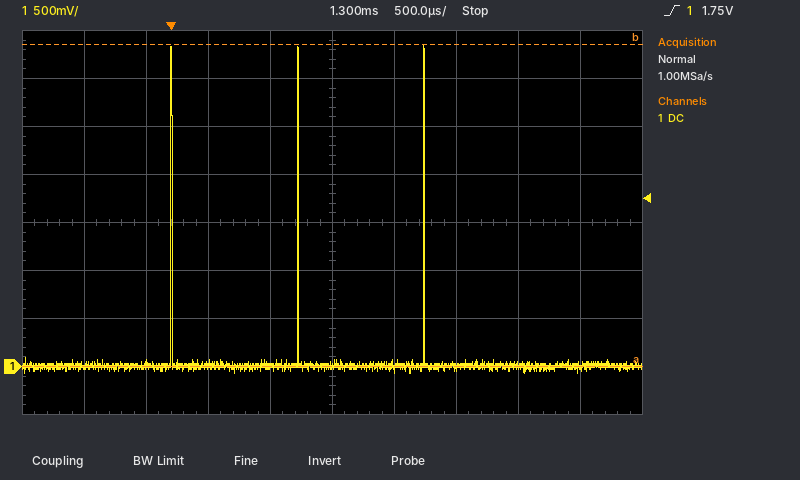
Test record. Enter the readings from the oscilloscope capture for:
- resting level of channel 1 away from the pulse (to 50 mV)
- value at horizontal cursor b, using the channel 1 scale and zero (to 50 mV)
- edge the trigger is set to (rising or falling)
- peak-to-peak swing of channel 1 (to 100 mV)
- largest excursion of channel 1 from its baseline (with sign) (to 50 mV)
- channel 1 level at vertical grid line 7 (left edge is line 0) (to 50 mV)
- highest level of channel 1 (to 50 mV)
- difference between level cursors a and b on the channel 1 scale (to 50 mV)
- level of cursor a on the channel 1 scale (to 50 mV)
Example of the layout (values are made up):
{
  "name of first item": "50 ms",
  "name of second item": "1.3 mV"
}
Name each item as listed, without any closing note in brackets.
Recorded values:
{
  "resting level of channel 1 away from the pulse": "0 mV",
  "value at horizontal cursor b, using the channel 1 scale and zero": "3.35 V",
  "edge the trigger is set to": "rising",
  "peak-to-peak swing of channel 1": "3.40 V",
  "largest excursion of channel 1 from its baseline (with sign)": "+3.35 V",
  "channel 1 level at vertical grid line 7 (left edge is line 0)": "0 mV",
  "highest level of channel 1": "3.35 V",
  "difference between level cursors a and b on the channel 1 scale": "3.35 V",
  "level of cursor a on the channel 1 scale": "0 mV"
}
